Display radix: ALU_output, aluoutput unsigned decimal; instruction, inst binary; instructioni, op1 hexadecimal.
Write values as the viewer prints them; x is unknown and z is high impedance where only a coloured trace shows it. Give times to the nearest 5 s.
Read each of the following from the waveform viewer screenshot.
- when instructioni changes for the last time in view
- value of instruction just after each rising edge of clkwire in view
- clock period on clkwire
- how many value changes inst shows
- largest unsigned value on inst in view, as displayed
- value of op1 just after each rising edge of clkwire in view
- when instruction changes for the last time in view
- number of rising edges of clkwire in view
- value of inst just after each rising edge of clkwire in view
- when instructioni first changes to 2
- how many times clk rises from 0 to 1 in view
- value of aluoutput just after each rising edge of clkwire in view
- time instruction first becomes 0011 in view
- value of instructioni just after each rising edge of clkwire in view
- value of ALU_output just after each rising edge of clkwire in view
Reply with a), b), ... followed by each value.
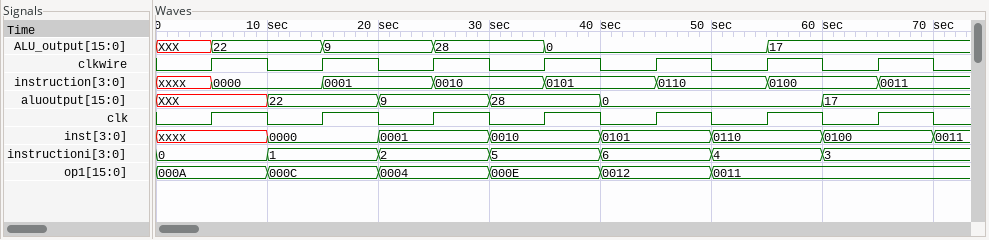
a) 60 s
b) 0000, 0001, 0010, 0101, 0110, 0100, 0011
c) 10 s
d) 7
e) 0110
f) 000A, 000C, 0004, 000E, 0012, 0011, 0011
g) 65 s
h) 7
i) xxxx, 0000, 0001, 0010, 0101, 0110, 0100
j) 20 s
k) 7
l) XXX, 22, 9, 28, 0, 0, 17
m) 65 s
n) 0, 1, 2, 5, 6, 4, 3
o) 22, 9, 28, 0, 0, 17, 17
